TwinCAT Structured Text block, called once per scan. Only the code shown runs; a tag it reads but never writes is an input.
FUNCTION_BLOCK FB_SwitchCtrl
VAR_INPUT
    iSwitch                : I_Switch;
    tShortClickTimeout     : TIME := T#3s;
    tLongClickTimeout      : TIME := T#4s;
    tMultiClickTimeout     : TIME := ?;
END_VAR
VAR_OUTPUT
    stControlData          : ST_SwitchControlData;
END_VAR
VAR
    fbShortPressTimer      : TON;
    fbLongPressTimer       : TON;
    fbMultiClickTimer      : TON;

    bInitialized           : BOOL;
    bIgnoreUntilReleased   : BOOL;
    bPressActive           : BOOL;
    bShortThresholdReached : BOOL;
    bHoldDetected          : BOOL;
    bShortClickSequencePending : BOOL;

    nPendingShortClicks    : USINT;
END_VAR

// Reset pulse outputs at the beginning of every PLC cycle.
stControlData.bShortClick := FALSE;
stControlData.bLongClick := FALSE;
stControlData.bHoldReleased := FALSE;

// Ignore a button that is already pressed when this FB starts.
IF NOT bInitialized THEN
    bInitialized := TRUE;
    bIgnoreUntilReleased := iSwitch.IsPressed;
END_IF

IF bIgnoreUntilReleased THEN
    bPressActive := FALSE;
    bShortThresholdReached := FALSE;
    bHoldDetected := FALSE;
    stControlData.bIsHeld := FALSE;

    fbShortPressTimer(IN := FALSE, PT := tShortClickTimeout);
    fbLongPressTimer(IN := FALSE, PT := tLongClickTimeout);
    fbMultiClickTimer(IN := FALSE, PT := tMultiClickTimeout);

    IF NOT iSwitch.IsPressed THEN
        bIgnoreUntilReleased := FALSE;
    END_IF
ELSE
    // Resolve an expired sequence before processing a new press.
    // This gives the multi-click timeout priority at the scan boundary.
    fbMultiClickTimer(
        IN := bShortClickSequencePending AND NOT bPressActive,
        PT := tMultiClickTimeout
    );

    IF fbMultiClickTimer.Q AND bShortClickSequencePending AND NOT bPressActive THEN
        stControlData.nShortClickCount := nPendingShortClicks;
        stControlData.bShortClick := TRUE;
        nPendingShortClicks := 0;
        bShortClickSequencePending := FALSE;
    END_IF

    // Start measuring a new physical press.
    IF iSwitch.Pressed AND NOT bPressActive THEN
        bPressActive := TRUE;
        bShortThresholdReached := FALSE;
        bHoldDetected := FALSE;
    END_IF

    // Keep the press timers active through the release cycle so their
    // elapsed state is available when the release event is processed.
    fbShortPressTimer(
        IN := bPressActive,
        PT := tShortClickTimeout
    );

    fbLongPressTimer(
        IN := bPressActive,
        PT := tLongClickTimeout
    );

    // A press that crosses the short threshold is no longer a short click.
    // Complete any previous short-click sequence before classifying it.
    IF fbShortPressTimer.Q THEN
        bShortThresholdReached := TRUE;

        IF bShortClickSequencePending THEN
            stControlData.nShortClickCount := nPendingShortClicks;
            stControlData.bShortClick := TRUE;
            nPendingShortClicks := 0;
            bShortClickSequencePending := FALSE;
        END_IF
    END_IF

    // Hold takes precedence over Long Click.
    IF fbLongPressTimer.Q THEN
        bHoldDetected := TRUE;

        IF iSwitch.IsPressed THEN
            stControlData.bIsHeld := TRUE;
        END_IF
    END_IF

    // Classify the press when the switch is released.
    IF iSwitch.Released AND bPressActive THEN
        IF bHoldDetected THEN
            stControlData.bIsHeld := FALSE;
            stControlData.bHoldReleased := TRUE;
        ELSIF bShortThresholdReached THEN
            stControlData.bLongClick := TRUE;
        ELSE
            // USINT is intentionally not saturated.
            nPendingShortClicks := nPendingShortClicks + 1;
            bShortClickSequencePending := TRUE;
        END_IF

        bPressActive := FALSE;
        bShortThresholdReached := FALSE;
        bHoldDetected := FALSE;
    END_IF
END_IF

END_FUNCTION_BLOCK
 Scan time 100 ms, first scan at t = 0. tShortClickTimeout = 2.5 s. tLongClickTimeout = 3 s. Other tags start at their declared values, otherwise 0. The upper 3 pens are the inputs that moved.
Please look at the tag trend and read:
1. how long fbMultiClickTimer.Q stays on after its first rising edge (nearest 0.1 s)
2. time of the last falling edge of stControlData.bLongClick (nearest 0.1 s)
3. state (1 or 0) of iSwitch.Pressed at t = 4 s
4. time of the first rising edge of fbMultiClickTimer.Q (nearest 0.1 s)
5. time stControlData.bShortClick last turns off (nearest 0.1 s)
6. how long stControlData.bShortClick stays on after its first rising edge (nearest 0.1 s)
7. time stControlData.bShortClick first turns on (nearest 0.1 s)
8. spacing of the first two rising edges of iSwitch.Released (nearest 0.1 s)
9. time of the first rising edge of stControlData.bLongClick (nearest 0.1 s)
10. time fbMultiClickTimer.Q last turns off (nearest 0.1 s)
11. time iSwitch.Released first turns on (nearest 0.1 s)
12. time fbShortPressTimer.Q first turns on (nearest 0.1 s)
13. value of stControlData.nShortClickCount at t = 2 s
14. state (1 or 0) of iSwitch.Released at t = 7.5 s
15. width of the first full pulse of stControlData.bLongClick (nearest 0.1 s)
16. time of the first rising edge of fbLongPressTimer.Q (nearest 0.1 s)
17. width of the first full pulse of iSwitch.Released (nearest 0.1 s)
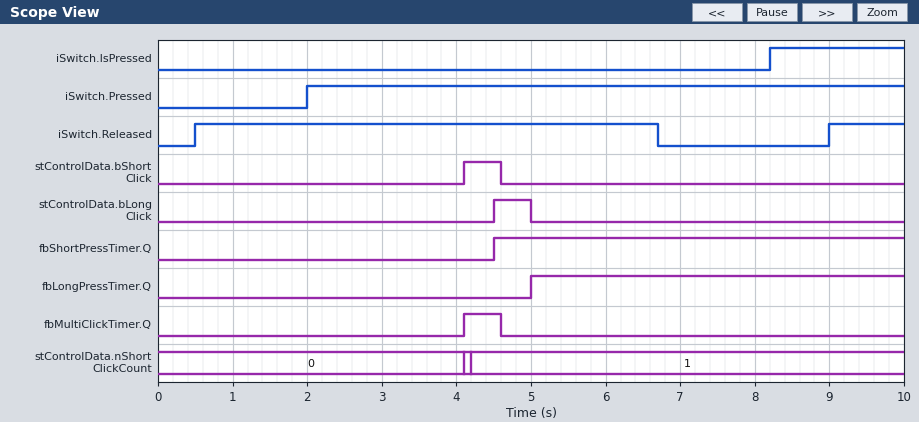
0.5 s
5.0 s
1
4.1 s
4.6 s
0.5 s
4.1 s
8.5 s
4.5 s
4.6 s
0.5 s
4.5 s
0
0
0.5 s
5.0 s
6.2 s
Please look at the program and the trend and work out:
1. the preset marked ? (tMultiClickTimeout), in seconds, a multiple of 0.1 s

2.0 s
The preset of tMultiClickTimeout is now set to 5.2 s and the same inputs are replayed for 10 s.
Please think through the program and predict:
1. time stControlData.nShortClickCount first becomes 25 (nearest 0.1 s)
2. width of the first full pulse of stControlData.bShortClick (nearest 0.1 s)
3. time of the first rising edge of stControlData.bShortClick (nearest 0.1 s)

4.5 s
0.1 s
4.5 s
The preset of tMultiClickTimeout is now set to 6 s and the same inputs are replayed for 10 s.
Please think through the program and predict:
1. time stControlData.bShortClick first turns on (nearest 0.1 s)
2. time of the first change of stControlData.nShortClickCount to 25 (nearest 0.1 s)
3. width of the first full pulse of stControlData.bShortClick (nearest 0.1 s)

4.5 s
4.5 s
0.1 s
